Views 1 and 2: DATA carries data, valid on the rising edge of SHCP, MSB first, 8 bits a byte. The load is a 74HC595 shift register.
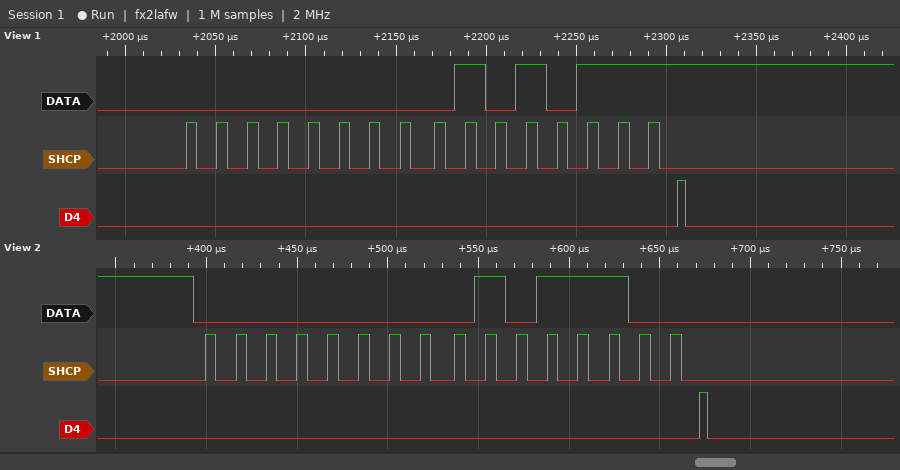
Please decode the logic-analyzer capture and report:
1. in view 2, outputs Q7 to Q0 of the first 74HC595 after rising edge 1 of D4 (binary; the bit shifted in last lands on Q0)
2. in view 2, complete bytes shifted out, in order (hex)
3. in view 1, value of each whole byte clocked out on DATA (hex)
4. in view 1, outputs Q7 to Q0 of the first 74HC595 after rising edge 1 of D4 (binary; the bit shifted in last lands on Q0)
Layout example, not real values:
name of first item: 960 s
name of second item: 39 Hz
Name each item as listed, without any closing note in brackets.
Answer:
in view 2, outputs Q7 to Q0 of the first 74HC595 after rising edge 1 of D4: 01011100
in view 2, complete bytes shifted out, in order: 00 5C
in view 1, value of each whole byte clocked out on DATA: 00 57
in view 1, outputs Q7 to Q0 of the first 74HC595 after rising edge 1 of D4: 01010111
